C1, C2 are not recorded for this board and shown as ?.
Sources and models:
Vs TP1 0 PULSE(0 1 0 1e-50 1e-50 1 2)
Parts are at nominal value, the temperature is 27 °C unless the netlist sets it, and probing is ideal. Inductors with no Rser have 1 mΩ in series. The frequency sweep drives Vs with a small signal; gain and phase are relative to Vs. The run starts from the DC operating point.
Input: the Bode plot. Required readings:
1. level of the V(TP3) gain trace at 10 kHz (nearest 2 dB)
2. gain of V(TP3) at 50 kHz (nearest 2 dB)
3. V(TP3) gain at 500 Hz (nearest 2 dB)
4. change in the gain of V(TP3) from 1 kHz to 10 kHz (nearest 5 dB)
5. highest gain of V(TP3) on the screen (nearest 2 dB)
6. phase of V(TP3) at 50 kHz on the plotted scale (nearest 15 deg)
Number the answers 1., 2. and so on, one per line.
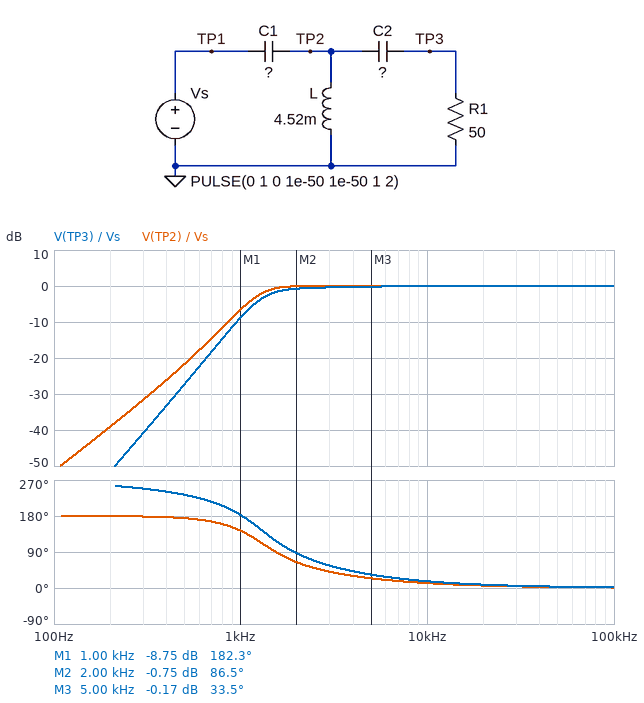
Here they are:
1. 0 dB
2. 0 dB
3. -28 dB
4. 10 dB
5. 0 dB
6. 0 deg
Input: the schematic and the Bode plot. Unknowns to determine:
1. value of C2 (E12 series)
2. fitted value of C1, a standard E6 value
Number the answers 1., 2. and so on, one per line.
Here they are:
1. 3.9 µF
2. 1.5 µF
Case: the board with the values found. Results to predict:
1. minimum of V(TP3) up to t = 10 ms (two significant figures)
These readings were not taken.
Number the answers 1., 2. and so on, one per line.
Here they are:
1. -300 mV
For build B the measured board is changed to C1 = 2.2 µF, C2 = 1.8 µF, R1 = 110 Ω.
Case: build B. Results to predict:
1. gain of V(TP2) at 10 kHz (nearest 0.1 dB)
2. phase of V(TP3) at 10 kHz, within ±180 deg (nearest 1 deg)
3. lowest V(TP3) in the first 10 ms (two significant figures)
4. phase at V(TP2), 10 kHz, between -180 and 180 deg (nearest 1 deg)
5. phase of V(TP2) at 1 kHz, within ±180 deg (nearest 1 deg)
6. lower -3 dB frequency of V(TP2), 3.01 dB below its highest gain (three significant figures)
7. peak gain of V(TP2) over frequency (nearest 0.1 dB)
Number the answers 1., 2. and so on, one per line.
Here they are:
1. 0.2 dB
2. 8 deg
3. -540 mV
4. 4 deg
5. 162 deg
6. 1.28 kHz
7. 9.3 dB
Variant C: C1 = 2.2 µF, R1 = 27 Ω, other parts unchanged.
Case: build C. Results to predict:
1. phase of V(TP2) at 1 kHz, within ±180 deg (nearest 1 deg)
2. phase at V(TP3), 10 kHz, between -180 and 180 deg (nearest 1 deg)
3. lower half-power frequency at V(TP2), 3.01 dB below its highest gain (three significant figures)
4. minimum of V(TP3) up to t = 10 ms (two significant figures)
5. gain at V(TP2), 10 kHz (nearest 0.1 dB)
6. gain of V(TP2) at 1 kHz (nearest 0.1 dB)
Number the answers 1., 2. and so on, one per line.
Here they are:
1. 111 deg
2. 23 deg
3. 891 Hz
4. -200 mV
5. -0.4 dB
6. 1.2 dB
